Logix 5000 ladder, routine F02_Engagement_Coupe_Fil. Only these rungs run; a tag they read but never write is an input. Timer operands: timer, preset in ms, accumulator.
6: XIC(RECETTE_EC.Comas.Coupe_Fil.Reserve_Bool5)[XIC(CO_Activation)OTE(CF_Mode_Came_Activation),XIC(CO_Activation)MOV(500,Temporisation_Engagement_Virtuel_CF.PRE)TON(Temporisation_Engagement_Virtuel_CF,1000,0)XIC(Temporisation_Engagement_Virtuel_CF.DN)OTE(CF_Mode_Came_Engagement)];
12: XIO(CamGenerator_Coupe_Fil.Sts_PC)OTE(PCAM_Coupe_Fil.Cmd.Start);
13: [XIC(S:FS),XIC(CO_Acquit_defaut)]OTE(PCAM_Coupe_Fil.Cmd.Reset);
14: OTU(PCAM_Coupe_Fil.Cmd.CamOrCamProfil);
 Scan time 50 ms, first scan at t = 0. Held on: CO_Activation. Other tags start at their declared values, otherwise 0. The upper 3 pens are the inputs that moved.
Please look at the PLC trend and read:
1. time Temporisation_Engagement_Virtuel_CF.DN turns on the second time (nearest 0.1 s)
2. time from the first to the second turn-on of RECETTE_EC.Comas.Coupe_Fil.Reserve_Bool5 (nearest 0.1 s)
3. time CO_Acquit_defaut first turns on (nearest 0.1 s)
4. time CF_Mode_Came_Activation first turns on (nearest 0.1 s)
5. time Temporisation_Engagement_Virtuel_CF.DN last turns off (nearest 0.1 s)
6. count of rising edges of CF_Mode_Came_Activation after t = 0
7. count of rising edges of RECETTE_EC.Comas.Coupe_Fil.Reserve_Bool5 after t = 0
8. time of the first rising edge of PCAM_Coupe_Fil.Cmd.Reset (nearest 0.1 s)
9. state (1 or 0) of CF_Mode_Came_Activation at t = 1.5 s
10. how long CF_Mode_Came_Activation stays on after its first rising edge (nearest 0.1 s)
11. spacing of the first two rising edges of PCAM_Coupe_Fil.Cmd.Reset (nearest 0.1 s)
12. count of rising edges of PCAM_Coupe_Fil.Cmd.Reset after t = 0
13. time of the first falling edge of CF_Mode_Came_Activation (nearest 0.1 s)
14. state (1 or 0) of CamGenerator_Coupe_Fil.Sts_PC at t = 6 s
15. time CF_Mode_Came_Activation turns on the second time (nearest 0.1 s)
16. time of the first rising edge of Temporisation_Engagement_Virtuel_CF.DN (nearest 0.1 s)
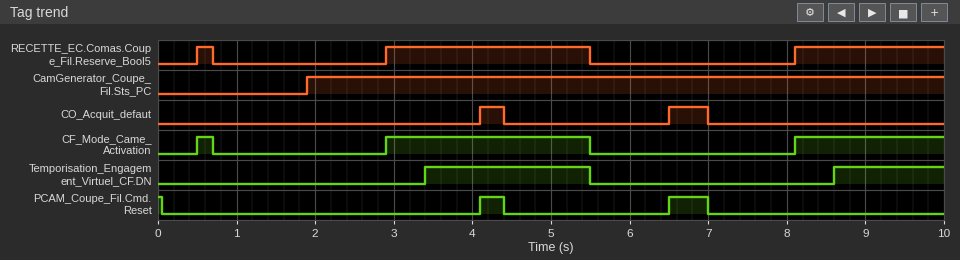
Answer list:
8.6 s
2.4 s
4.1 s
0.5 s
5.5 s
3
3
4.1 s
0
0.2 s
2.4 s
2
0.7 s
1
2.9 s
3.4 s
